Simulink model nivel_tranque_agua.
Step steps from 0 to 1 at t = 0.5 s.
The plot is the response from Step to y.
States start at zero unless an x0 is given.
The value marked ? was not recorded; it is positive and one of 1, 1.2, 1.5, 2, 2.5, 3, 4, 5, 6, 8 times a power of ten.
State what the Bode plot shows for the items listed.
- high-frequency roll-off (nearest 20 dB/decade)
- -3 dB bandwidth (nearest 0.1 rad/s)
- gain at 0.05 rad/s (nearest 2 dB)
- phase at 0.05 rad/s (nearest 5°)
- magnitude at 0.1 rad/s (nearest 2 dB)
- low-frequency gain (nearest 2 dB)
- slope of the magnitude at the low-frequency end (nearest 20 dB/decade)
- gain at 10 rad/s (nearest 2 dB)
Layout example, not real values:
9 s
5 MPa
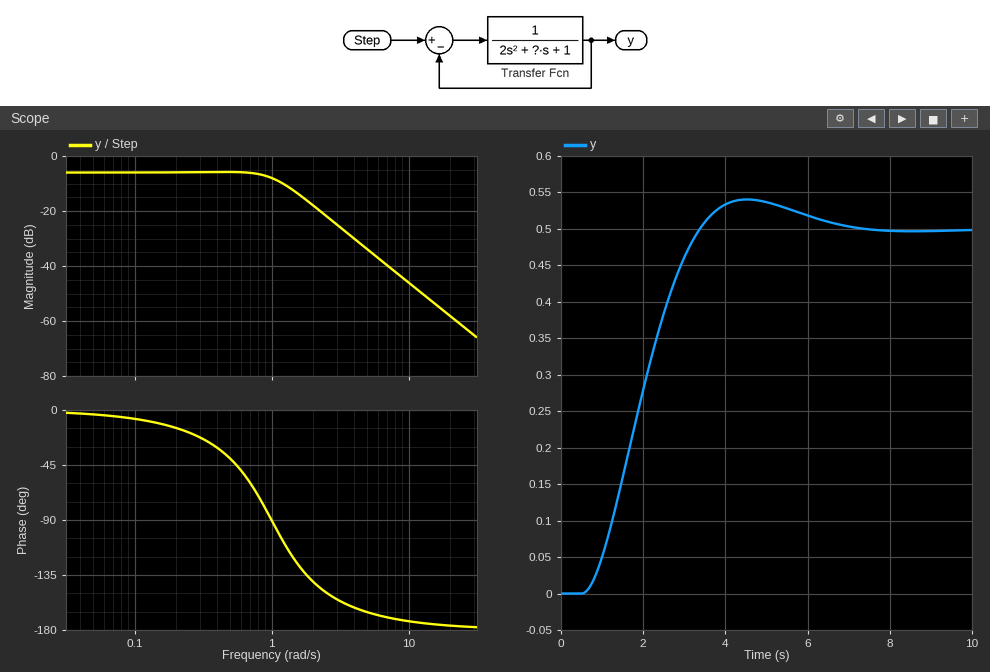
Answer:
-40 dB/decade
1.1 rad/s
-6 dB
-5°
-6 dB
-6 dB
0 dB/decade
-46 dB
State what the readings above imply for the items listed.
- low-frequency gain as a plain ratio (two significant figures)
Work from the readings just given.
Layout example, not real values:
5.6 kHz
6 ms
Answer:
0.50
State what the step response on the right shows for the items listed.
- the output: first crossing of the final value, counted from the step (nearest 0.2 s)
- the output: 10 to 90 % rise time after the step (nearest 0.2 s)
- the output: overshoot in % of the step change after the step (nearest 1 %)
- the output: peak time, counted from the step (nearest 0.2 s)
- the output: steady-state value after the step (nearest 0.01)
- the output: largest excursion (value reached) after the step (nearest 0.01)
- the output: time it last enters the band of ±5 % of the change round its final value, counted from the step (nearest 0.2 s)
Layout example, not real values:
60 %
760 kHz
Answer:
2.8 s
2.0 s
8 %
4.0 s
0.50
0.54
5.2 s
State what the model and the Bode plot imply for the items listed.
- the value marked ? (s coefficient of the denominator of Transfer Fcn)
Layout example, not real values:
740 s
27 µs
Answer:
2.5
